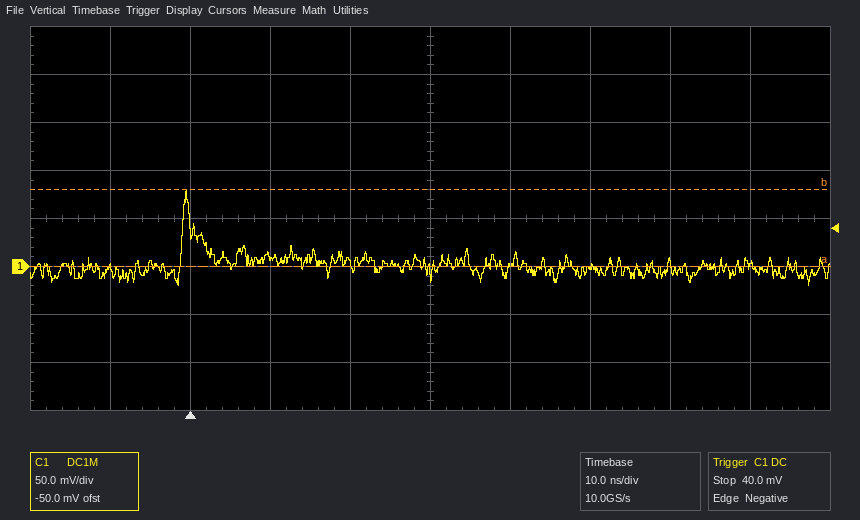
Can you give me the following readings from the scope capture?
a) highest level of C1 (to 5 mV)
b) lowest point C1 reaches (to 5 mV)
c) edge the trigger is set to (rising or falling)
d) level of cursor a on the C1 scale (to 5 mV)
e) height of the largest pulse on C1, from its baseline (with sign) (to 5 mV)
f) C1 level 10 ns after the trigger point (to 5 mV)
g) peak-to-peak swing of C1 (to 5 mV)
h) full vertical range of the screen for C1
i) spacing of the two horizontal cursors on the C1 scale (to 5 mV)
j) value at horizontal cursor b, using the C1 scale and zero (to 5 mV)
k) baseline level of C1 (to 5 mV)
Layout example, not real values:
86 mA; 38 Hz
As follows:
80 mV; -20 mV; falling; 0 mV; +80 mV; 10 mV; 100 mV; 400 mV; 80 mV; 80 mV; 0 mV
